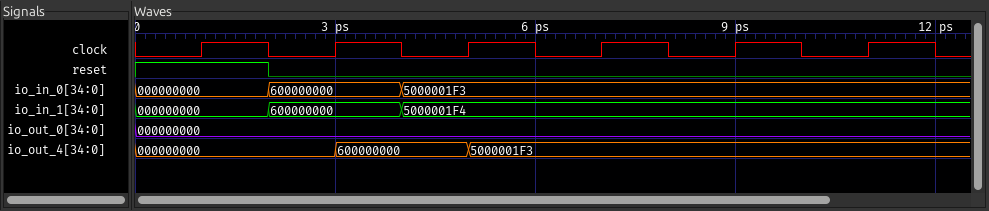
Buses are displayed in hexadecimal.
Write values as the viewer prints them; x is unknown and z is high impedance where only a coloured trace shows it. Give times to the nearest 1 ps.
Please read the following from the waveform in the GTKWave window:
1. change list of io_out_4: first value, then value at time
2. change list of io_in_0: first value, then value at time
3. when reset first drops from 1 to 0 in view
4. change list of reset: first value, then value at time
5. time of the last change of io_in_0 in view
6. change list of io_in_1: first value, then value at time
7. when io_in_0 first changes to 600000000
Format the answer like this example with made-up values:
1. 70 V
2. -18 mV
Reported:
1. 000000000, 600000000 at 3 ps, 5000001F3 at 5 ps
2. 000000000, 600000000 at 2 ps, 5000001F3 at 4 ps
3. 2 ps
4. 1, 0 at 2 ps
5. 4 ps
6. 000000000, 600000000 at 2 ps, 5000001F4 at 4 ps
7. 2 ps
